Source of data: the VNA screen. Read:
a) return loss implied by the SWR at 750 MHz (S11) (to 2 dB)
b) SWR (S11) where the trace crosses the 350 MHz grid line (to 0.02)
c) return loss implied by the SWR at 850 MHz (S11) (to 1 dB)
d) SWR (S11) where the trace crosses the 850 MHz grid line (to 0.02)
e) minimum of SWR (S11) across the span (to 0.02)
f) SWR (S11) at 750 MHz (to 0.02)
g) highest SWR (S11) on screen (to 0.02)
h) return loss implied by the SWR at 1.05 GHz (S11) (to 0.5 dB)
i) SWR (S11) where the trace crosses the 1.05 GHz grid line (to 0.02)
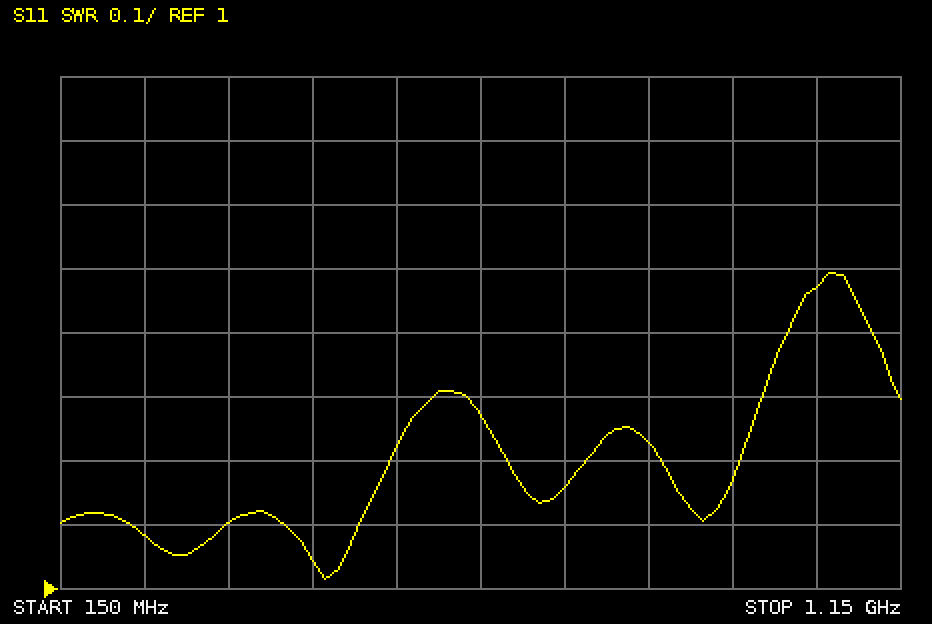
22 dB
1.10
20 dB
1.22
1.02
1.16
1.50
14.5 dB
1.48
